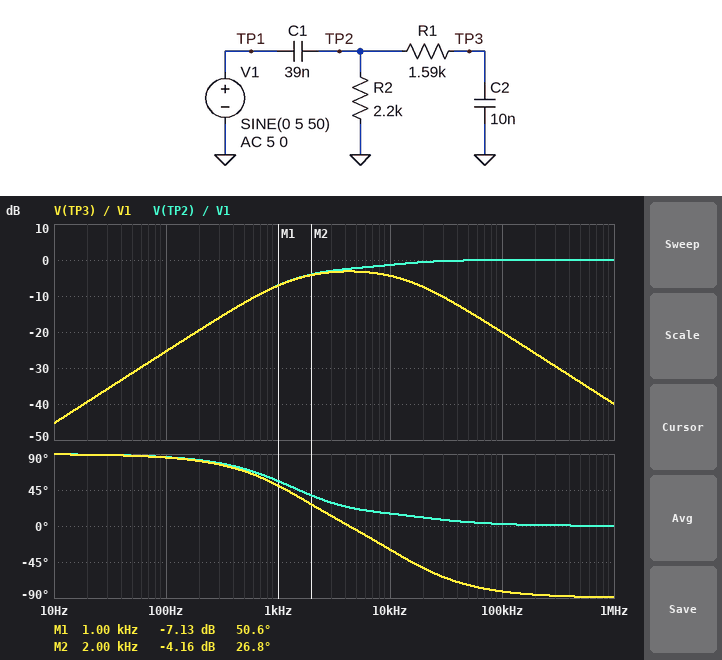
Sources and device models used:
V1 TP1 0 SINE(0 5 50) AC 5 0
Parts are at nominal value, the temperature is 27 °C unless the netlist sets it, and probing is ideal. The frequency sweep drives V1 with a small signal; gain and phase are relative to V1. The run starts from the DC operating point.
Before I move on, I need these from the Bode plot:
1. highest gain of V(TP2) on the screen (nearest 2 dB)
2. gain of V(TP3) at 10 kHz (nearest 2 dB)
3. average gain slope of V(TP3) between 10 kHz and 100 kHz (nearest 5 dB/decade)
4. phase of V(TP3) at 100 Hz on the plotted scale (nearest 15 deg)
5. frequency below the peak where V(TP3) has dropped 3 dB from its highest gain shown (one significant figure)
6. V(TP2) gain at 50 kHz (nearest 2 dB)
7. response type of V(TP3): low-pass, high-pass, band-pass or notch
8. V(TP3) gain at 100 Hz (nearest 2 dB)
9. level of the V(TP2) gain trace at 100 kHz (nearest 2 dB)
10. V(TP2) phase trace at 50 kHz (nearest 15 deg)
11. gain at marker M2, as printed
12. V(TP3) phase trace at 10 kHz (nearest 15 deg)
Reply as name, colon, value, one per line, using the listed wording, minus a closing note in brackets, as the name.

highest gain of V(TP2) on the screen: 0 dB
gain of V(TP3) at 10 kHz: -4 dB
average gain slope of V(TP3) between 10 kHz and 100 kHz: -15 dB/decade
phase of V(TP3) at 100 Hz on the plotted scale: 90 deg
frequency below the peak where V(TP3) has dropped 3 dB from its highest gain shown: 1 kHz
V(TP2) gain at 50 kHz: 0 dB
response type of V(TP3): low-pass, high-pass, band-pass or notch: band-pass
V(TP3) gain at 100 Hz: -26 dB
level of the V(TP2) gain trace at 100 kHz: 0 dB
V(TP2) phase trace at 50 kHz: 0 deg
gain at marker M2, as printed: -4.16 dB
V(TP3) phase trace at 10 kHz: -30 deg
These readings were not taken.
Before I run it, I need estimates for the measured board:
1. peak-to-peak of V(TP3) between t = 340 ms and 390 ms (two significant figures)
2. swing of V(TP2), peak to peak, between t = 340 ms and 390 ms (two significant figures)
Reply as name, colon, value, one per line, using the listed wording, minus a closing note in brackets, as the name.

peak-to-peak of V(TP3) between t = 340 ms and 390 ms: 270 mV
swing of V(TP2), peak to peak, between t = 340 ms and 390 ms: 270 mV
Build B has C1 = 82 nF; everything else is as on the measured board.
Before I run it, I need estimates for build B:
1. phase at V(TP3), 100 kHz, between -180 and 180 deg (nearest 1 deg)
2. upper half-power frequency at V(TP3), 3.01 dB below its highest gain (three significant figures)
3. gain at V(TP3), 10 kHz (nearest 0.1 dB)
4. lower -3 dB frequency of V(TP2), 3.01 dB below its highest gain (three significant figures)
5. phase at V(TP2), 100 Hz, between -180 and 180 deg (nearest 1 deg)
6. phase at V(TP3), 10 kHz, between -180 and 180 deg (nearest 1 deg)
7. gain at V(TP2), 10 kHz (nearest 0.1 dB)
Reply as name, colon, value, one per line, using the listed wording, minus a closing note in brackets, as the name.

phase at V(TP3), 100 kHz, between -180 and 180 deg: -83 deg
upper half-power frequency at V(TP3), 3.01 dB below its highest gain: 12.8 kHz
gain at V(TP3), 10 kHz: -3.6 dB
lower -3 dB frequency of V(TP2), 3.01 dB below its highest gain: 1.04 kHz
phase at V(TP2), 100 Hz, between -180 and 180 deg: 83 deg
phase at V(TP3), 10 kHz, between -180 and 180 deg: -37 deg
gain at V(TP2), 10 kHz: -0.6 dB
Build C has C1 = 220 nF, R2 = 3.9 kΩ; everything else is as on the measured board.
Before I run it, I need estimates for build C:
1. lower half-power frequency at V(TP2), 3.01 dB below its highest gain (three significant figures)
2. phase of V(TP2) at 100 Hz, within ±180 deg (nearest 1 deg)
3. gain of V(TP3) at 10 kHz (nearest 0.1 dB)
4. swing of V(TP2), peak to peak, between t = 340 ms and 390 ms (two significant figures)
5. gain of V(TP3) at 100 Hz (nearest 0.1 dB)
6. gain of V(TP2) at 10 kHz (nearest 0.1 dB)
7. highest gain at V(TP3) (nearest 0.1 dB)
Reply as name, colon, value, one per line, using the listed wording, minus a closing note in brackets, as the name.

lower half-power frequency at V(TP2), 3.01 dB below its highest gain: 195 Hz
phase of V(TP2) at 100 Hz, within ±180 deg: 61 deg
gain of V(TP3) at 10 kHz: -3.2 dB
swing of V(TP2), peak to peak, between t = 340 ms and 390 ms: 2.6 V
gain of V(TP3) at 100 Hz: -6.6 dB
gain of V(TP2) at 10 kHz: -0.2 dB
highest gain at V(TP3): -0.5 dB
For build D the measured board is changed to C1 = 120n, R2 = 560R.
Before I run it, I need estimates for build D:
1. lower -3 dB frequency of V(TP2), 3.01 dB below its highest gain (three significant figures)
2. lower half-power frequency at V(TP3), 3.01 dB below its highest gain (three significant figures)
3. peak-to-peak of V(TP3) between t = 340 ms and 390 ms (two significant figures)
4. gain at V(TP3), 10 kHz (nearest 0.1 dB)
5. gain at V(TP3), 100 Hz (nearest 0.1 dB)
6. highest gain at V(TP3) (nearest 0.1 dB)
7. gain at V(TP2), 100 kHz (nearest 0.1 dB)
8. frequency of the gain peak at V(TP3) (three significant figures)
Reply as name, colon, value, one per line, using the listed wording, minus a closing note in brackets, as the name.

lower -3 dB frequency of V(TP2), 3.01 dB below its highest gain: 2.65 kHz
lower half-power frequency at V(TP3), 3.01 dB below its highest gain: 1.60 kHz
peak-to-peak of V(TP3) between t = 340 ms and 390 ms: 210 mV
gain at V(TP3), 10 kHz: -3.7 dB
gain at V(TP3), 100 Hz: -27.5 dB
highest gain at V(TP3): -2.4 dB
gain at V(TP2), 100 kHz: 0 dB
frequency of the gain peak at V(TP3): 4.87 kHz
